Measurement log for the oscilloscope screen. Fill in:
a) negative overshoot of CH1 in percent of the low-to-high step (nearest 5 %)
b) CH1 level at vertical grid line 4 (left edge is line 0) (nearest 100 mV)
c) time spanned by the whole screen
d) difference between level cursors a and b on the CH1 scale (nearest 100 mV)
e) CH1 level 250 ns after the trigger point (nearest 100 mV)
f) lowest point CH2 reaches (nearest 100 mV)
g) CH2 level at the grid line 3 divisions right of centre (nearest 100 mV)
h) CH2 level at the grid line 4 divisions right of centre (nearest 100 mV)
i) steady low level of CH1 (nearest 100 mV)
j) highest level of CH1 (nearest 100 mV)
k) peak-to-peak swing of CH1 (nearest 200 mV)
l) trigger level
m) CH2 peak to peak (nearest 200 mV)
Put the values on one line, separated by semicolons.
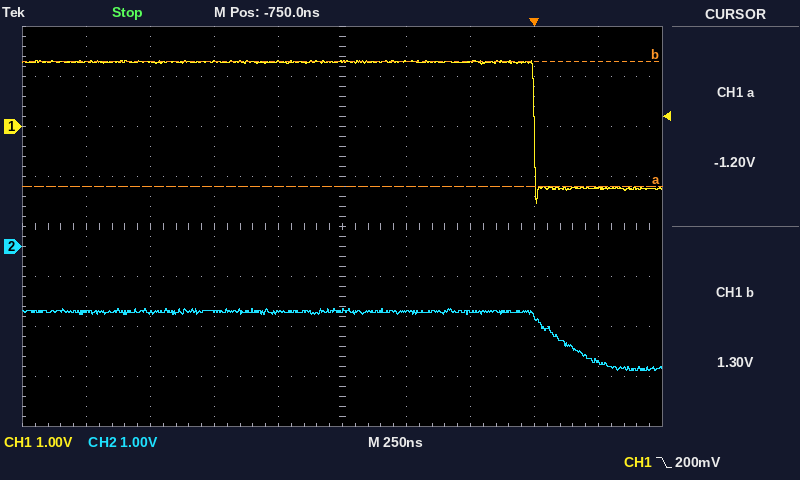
10 %; 1.3 V; 2.5 µs; 2.5 V; -1.2 V; -2.5 V; -1.4 V; -2.3 V; -1.2 V; 1.3 V; 2.8 V; 200 mV; 1.2 V
